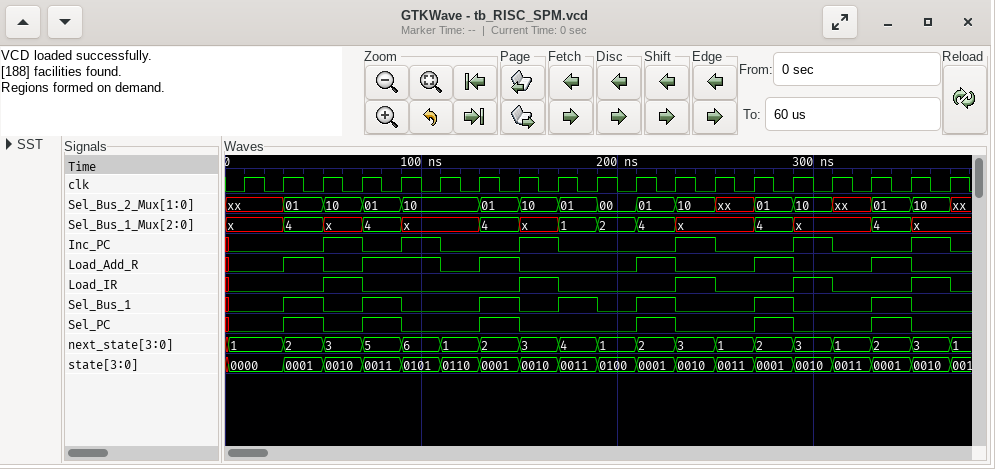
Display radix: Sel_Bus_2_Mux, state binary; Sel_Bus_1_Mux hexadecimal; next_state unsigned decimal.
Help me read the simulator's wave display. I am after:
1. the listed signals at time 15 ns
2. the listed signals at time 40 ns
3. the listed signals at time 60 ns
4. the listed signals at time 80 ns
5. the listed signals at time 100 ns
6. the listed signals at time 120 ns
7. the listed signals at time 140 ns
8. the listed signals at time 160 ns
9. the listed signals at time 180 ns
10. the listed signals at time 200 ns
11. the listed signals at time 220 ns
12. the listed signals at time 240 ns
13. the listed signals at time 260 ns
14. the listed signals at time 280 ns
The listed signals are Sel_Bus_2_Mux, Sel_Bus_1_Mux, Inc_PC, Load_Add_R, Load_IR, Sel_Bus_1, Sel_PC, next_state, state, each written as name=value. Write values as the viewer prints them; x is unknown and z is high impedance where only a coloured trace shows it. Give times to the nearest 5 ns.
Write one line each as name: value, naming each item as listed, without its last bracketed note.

the listed signals at time 15 ns: Sel_Bus_2_Mux=xx, Sel_Bus_1_Mux=x, Inc_PC=0, Load_Add_R=0, Load_IR=0, Sel_Bus_1=0, Sel_PC=0, next_state=1, state=0000
the listed signals at time 40 ns: Sel_Bus_2_Mux=01, Sel_Bus_1_Mux=4, Inc_PC=0, Load_Add_R=1, Load_IR=0, Sel_Bus_1=1, Sel_PC=1, next_state=2, state=0001
the listed signals at time 60 ns: Sel_Bus_2_Mux=10, Sel_Bus_1_Mux=x, Inc_PC=1, Load_Add_R=0, Load_IR=1, Sel_Bus_1=0, Sel_PC=0, next_state=3, state=0010
the listed signals at time 80 ns: Sel_Bus_2_Mux=01, Sel_Bus_1_Mux=4, Inc_PC=0, Load_Add_R=1, Load_IR=0, Sel_Bus_1=1, Sel_PC=1, next_state=5, state=0011
the listed signals at time 100 ns: Sel_Bus_2_Mux=10, Sel_Bus_1_Mux=x, Inc_PC=1, Load_Add_R=1, Load_IR=0, Sel_Bus_1=0, Sel_PC=0, next_state=6, state=0101
the listed signals at time 120 ns: Sel_Bus_2_Mux=10, Sel_Bus_1_Mux=x, Inc_PC=0, Load_Add_R=0, Load_IR=0, Sel_Bus_1=0, Sel_PC=0, next_state=1, state=0110
the listed signals at time 140 ns: Sel_Bus_2_Mux=01, Sel_Bus_1_Mux=4, Inc_PC=0, Load_Add_R=1, Load_IR=0, Sel_Bus_1=1, Sel_PC=1, next_state=2, state=0001
the listed signals at time 160 ns: Sel_Bus_2_Mux=10, Sel_Bus_1_Mux=x, Inc_PC=1, Load_Add_R=0, Load_IR=1, Sel_Bus_1=0, Sel_PC=0, next_state=3, state=0010
the listed signals at time 180 ns: Sel_Bus_2_Mux=01, Sel_Bus_1_Mux=1, Inc_PC=0, Load_Add_R=0, Load_IR=0, Sel_Bus_1=1, Sel_PC=0, next_state=4, state=0011
the listed signals at time 200 ns: Sel_Bus_2_Mux=00, Sel_Bus_1_Mux=2, Inc_PC=0, Load_Add_R=0, Load_IR=0, Sel_Bus_1=0, Sel_PC=0, next_state=1, state=0100
the listed signals at time 220 ns: Sel_Bus_2_Mux=01, Sel_Bus_1_Mux=4, Inc_PC=0, Load_Add_R=1, Load_IR=0, Sel_Bus_1=1, Sel_PC=1, next_state=2, state=0001
the listed signals at time 240 ns: Sel_Bus_2_Mux=10, Sel_Bus_1_Mux=x, Inc_PC=1, Load_Add_R=0, Load_IR=1, Sel_Bus_1=0, Sel_PC=0, next_state=3, state=0010
the listed signals at time 260 ns: Sel_Bus_2_Mux=xx, Sel_Bus_1_Mux=x, Inc_PC=0, Load_Add_R=0, Load_IR=0, Sel_Bus_1=0, Sel_PC=0, next_state=1, state=0011
the listed signals at time 280 ns: Sel_Bus_2_Mux=01, Sel_Bus_1_Mux=4, Inc_PC=0, Load_Add_R=1, Load_IR=0, Sel_Bus_1=1, Sel_PC=1, next_state=2, state=0001
